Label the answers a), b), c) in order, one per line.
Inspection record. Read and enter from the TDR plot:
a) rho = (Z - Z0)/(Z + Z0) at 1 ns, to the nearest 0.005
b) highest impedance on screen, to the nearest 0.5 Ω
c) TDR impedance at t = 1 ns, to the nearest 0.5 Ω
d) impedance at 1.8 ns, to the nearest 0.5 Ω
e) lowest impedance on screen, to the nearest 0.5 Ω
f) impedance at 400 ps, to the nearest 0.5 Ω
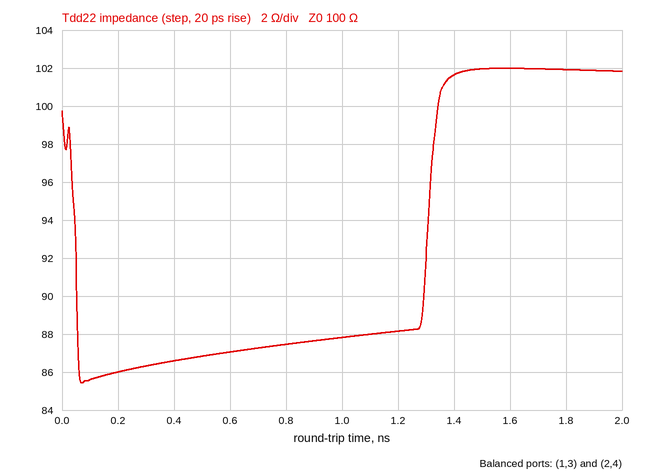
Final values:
a) -0.065
b) 102.0 Ω
c) 88.0 Ω
d) 102.0 Ω
e) 85.5 Ω
f) 86.5 Ω
